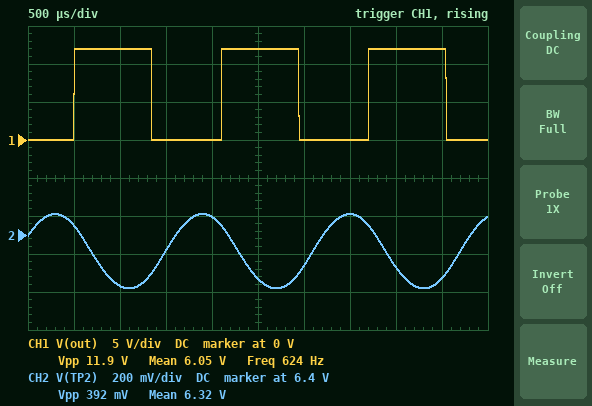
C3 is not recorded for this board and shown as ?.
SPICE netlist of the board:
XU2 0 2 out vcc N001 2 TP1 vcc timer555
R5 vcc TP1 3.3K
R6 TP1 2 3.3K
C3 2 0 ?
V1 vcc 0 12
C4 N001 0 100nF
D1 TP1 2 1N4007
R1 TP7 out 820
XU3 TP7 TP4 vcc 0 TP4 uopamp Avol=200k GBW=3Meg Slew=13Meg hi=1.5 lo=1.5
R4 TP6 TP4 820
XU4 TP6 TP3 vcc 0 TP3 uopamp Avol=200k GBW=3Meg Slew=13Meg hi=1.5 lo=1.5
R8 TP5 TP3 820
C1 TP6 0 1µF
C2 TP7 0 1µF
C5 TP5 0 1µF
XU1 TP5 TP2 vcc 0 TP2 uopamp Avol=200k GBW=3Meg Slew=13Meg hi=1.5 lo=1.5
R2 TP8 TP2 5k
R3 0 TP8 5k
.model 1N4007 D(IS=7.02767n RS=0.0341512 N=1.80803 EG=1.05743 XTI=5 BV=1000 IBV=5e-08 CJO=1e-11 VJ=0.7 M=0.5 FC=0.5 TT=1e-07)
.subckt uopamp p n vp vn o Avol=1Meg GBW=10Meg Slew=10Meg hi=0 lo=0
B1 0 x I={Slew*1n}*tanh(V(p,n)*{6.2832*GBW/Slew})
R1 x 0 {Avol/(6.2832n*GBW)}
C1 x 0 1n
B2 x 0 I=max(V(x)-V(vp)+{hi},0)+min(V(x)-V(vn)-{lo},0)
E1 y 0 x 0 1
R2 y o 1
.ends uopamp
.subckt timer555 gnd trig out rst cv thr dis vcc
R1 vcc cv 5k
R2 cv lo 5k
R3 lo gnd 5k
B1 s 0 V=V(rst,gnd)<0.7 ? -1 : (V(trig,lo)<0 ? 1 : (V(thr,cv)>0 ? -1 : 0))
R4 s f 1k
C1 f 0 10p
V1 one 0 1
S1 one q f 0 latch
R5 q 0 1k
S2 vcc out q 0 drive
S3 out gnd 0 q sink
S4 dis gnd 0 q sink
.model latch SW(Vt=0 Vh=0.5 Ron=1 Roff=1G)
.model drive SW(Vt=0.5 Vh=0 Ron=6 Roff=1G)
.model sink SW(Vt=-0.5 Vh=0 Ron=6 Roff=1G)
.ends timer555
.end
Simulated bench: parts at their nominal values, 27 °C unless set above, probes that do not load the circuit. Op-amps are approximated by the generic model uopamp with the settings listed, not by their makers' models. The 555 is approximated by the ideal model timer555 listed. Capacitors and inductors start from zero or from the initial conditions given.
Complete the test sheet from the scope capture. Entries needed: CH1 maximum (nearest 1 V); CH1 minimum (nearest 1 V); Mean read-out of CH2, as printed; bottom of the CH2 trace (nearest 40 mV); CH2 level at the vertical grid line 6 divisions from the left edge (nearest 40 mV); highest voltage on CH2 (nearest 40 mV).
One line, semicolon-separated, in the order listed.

12 V; 0 V; 6.32 V; 6.12 V; 6.24 V; 6.52 V
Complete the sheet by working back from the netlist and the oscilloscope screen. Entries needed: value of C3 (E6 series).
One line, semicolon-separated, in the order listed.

330 nF
